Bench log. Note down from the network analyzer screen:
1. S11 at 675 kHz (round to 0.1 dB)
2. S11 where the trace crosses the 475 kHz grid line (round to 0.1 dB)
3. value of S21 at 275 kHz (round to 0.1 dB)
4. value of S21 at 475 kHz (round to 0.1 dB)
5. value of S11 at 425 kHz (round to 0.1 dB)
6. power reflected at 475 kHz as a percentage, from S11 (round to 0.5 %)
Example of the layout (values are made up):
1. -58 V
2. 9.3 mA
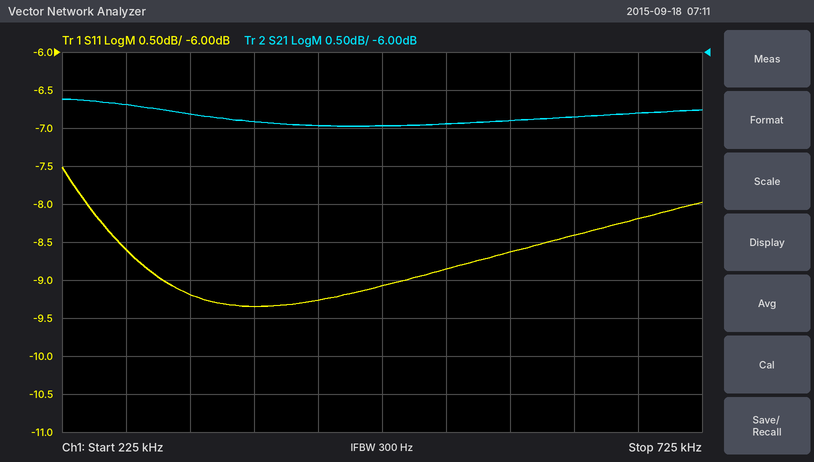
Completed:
1. -8.2 dB
2. -9.1 dB
3. -6.7 dB
4. -7.0 dB
5. -9.3 dB
6. 12.5 %
